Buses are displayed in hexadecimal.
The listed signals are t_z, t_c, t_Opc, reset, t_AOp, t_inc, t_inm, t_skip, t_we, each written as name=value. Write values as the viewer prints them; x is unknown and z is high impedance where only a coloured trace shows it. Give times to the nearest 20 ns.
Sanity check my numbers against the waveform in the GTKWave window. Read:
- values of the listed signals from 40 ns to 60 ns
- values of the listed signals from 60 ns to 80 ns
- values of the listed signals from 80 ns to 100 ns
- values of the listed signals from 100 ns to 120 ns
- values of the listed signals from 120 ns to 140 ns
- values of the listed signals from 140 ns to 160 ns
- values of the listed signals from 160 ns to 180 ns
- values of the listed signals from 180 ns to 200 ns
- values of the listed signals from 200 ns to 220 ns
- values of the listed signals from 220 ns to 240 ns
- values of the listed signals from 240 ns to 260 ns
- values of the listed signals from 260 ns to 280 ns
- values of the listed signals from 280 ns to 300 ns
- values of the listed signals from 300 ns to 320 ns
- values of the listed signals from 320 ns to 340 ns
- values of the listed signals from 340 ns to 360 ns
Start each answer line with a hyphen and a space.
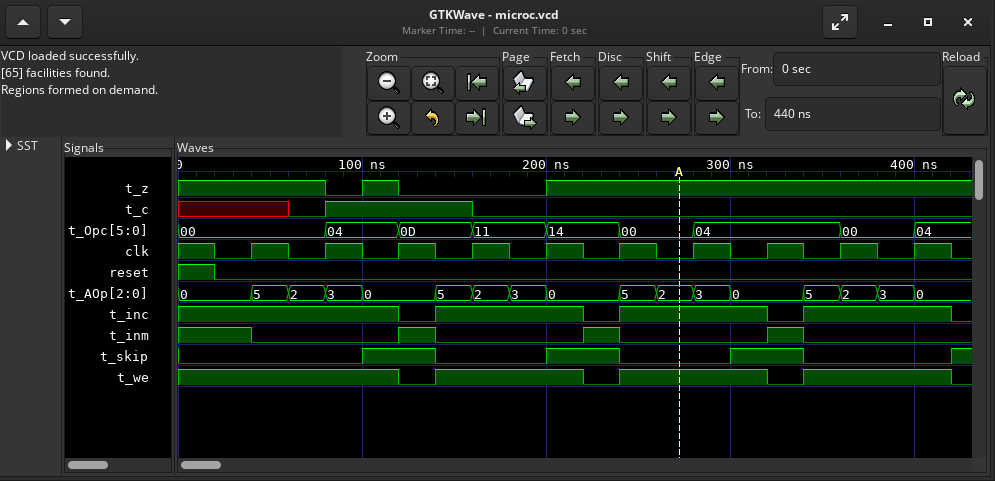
- t_z=1, t_c=x, t_Opc=00, reset=0, t_AOp=5, t_inc=1, t_inm=0, t_skip=0, t_we=1
- t_z=1, t_c=0, t_Opc=00, reset=0, t_AOp=2, t_inc=1, t_inm=0, t_skip=0, t_we=1
- t_z=0, t_c=1, t_Opc=04, reset=0, t_AOp=3, t_inc=1, t_inm=0, t_skip=0, t_we=1
- t_z=1, t_c=1, t_Opc=04, reset=0, t_AOp=0, t_inc=1, t_inm=0, t_skip=1, t_we=1
- t_z=0, t_c=1, t_Opc=0D, reset=0, t_AOp=0, t_inc=0, t_inm=1, t_skip=1, t_we=0
- t_z=0, t_c=1, t_Opc=0D, reset=0, t_AOp=5, t_inc=1, t_inm=0, t_skip=0, t_we=1
- t_z=0, t_c=0, t_Opc=11, reset=0, t_AOp=2, t_inc=1, t_inm=0, t_skip=0, t_we=1
- t_z=0, t_c=0, t_Opc=11, reset=0, t_AOp=3, t_inc=1, t_inm=0, t_skip=0, t_we=1
- t_z=1, t_c=0, t_Opc=14, reset=0, t_AOp=0, t_inc=1, t_inm=0, t_skip=1, t_we=1
- t_z=1, t_c=0, t_Opc=14, reset=0, t_AOp=0, t_inc=0, t_inm=1, t_skip=1, t_we=0
- t_z=1, t_c=0, t_Opc=00, reset=0, t_AOp=5, t_inc=1, t_inm=0, t_skip=0, t_we=1
- t_z=1, t_c=0, t_Opc=00, reset=0, t_AOp=2, t_inc=1, t_inm=0, t_skip=0, t_we=1
- t_z=1, t_c=0, t_Opc=04, reset=0, t_AOp=3, t_inc=1, t_inm=0, t_skip=0, t_we=1
- t_z=1, t_c=0, t_Opc=04, reset=0, t_AOp=0, t_inc=1, t_inm=0, t_skip=1, t_we=1
- t_z=1, t_c=0, t_Opc=04, reset=0, t_AOp=0, t_inc=0, t_inm=1, t_skip=1, t_we=0
- t_z=1, t_c=0, t_Opc=04, reset=0, t_AOp=5, t_inc=1, t_inm=0, t_skip=0, t_we=1
